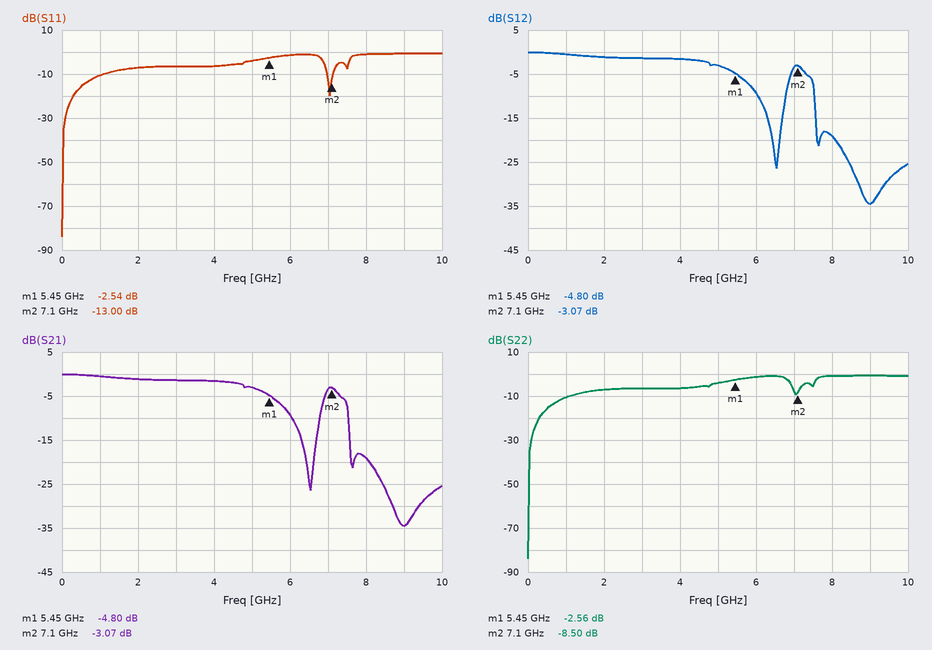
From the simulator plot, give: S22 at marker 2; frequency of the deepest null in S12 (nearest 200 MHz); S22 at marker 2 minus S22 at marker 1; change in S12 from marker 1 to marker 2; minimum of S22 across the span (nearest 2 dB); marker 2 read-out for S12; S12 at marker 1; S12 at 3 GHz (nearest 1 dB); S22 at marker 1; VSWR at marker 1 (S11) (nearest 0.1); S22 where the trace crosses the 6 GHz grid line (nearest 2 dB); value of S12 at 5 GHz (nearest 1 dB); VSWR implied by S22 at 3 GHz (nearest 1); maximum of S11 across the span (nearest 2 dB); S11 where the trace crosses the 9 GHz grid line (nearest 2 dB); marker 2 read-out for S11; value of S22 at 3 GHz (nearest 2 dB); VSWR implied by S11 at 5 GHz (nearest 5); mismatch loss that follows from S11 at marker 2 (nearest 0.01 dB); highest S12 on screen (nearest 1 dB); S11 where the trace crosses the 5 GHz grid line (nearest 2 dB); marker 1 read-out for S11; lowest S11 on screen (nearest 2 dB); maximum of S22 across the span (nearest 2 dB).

-8.50 dB
9.0 GHz
-5.94 dB
1.73 dB
-84 dB
-3.07 dB
-4.80 dB
-1 dB
-2.56 dB
6.9
-2 dB
-3 dB
3
0 dB
0 dB
-13.00 dB
-6 dB
5
0.22 dB
0 dB
-4 dB
-2.54 dB
-84 dB
0 dB
